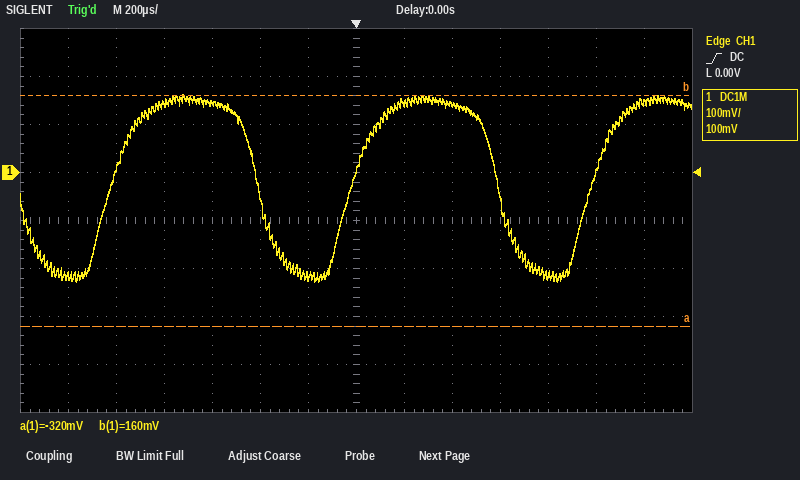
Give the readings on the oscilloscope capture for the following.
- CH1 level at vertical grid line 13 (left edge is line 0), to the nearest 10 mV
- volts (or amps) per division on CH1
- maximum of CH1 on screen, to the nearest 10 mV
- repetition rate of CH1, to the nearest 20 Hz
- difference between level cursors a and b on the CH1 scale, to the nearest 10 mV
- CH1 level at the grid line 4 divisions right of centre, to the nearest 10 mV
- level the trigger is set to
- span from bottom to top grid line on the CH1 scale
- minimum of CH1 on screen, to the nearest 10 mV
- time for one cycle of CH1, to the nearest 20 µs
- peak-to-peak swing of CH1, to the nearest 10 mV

150 mV
100 mV
160 mV
1.00 kHz
480 mV
-210 mV
0.00 V
800 mV
-230 mV
1.00 ms
390 mV
